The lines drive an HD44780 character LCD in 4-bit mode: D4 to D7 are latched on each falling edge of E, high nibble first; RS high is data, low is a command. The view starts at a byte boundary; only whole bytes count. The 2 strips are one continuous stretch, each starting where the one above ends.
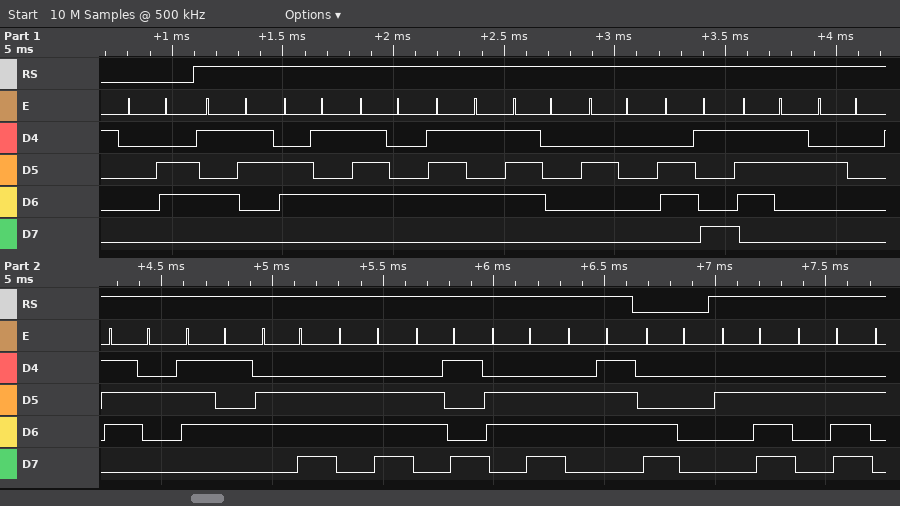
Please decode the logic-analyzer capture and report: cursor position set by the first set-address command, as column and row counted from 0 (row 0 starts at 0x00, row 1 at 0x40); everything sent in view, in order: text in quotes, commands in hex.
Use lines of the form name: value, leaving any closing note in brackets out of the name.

cursor position set by the first set-address command, as column and row counted from 0: column 0, row 1
everything sent in view, in order: text in quotes, commands in hex: 0x06 "Setup is running" 0xC0 ".."
